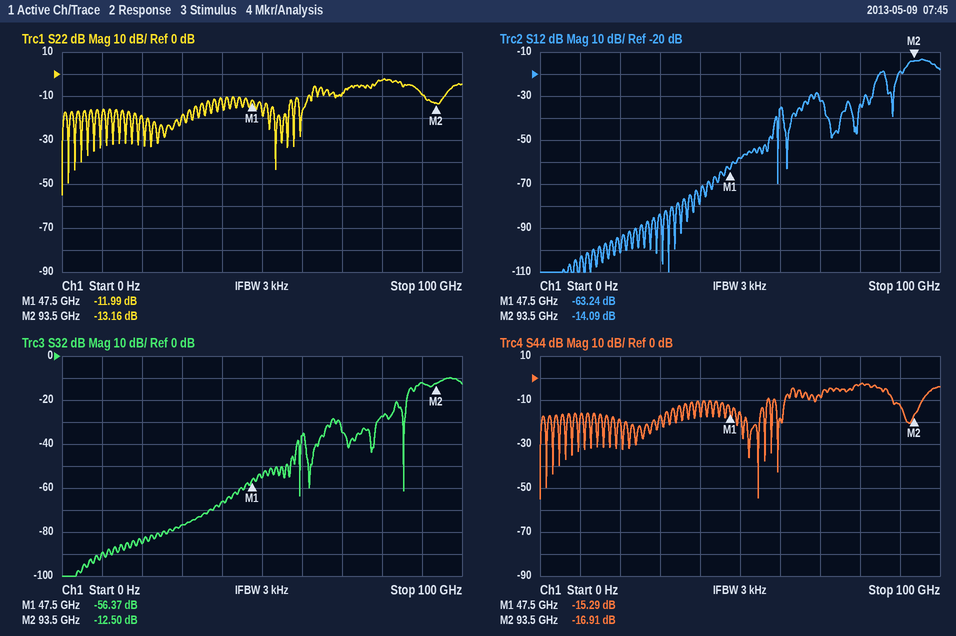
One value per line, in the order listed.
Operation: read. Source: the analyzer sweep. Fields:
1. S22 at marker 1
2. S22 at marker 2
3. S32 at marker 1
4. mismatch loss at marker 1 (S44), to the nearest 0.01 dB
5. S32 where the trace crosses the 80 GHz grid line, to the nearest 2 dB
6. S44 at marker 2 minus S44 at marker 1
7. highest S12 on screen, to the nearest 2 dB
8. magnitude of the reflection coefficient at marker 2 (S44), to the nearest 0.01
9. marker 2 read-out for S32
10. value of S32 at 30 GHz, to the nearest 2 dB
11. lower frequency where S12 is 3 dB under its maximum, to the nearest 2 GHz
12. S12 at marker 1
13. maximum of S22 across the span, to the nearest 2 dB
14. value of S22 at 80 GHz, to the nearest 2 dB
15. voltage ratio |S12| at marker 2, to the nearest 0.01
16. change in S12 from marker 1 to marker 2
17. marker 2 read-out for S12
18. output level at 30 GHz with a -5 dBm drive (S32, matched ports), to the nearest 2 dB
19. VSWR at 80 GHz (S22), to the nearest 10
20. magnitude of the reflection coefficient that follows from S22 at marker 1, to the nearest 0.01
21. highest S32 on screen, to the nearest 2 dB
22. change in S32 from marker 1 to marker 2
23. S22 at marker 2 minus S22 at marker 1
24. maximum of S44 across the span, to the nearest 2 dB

-11.99 dB
-13.16 dB
-56.37 dB
0.13 dB
-28 dB
-1.62 dB
-14 dB
0.14
-12.50 dB
-76 dB
92 GHz
-63.24 dB
-2 dB
-2 dB
0.20
49.15 dB
-14.09 dB
-82 dBm
10
0.25
-10 dB
43.87 dB
-1.17 dB
-2 dB
